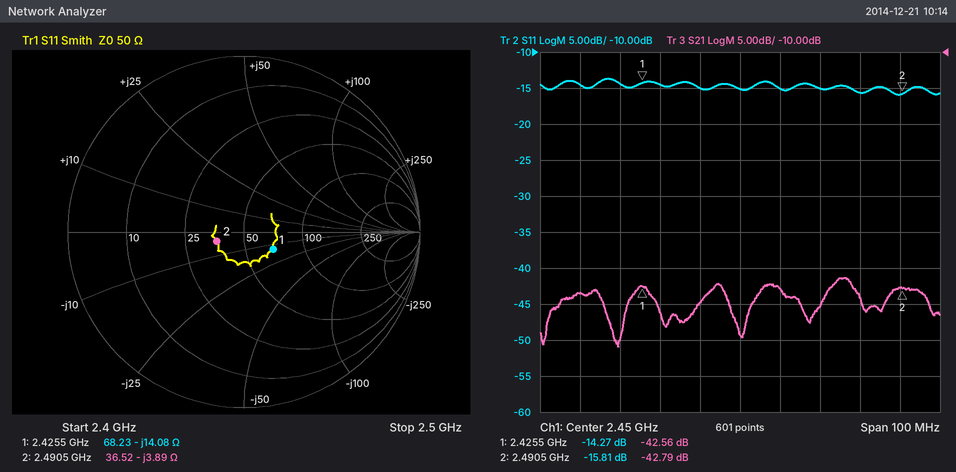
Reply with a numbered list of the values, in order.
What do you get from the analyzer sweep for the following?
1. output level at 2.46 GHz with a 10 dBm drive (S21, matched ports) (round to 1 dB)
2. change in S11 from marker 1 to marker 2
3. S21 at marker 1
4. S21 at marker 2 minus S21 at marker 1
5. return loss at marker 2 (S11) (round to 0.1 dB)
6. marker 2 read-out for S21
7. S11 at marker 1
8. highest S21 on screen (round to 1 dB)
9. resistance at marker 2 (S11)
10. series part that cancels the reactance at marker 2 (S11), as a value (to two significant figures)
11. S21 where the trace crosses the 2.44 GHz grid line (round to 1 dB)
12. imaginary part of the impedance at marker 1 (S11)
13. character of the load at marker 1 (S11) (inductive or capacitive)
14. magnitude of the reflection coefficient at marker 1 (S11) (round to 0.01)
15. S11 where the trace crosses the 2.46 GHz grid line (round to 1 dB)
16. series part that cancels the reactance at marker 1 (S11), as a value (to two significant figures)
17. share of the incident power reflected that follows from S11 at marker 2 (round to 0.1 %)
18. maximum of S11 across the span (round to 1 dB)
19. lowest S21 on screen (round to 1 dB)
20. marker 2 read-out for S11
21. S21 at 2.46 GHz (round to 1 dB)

1. -33 dBm
2. -1.54 dB
3. -42.56 dB
4. -0.23 dB
5. 15.8 dB
6. -42.79 dB
7. -14.27 dB
8. -41 dB
9. 36.52 Ω
10. 250 pH
11. -45 dB
12. -14.08 Ω
13. capacitive
14. 0.19
15. -15 dB
16. 920 pH
17. 2.6 %
18. -14 dB
19. -51 dB
20. -15.81 dB
21. -43 dB
